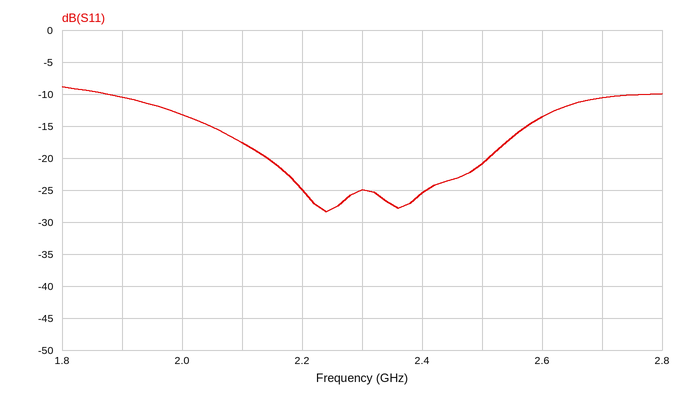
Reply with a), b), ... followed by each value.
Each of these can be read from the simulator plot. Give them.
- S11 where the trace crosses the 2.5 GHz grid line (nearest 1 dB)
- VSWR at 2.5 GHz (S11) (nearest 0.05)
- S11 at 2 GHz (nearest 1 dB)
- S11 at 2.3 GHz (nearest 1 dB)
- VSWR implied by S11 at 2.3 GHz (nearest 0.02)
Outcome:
a) -21 dB
b) 1.20
c) -13 dB
d) -25 dB
e) 1.12
